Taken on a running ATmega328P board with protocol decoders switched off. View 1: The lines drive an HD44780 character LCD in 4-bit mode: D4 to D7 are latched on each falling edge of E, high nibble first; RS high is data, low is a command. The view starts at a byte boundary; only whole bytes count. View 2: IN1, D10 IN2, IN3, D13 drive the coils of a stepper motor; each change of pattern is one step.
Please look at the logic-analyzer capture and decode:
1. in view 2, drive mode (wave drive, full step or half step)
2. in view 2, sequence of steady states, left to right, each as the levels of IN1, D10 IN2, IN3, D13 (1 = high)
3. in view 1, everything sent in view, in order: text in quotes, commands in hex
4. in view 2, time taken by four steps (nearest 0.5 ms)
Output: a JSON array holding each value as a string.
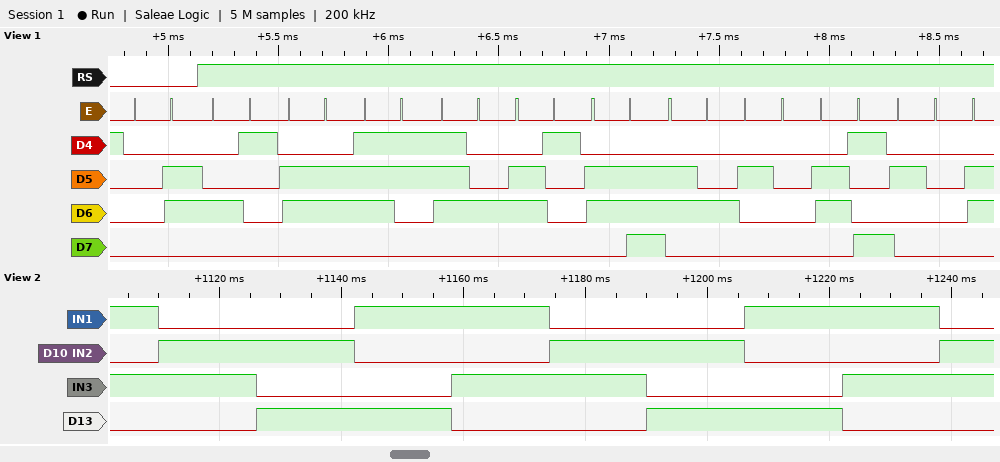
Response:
["full step", "1010 0110 0101 1001 1010 0110 0101 1001 1010 0110", "0x06 \"Afstand i \"", "64.0 ms"]
